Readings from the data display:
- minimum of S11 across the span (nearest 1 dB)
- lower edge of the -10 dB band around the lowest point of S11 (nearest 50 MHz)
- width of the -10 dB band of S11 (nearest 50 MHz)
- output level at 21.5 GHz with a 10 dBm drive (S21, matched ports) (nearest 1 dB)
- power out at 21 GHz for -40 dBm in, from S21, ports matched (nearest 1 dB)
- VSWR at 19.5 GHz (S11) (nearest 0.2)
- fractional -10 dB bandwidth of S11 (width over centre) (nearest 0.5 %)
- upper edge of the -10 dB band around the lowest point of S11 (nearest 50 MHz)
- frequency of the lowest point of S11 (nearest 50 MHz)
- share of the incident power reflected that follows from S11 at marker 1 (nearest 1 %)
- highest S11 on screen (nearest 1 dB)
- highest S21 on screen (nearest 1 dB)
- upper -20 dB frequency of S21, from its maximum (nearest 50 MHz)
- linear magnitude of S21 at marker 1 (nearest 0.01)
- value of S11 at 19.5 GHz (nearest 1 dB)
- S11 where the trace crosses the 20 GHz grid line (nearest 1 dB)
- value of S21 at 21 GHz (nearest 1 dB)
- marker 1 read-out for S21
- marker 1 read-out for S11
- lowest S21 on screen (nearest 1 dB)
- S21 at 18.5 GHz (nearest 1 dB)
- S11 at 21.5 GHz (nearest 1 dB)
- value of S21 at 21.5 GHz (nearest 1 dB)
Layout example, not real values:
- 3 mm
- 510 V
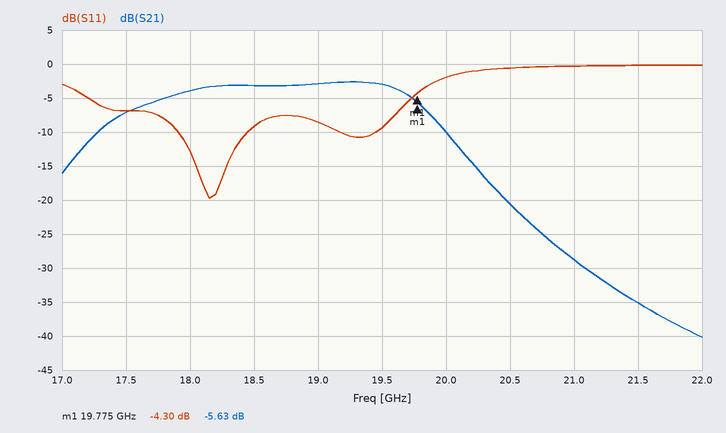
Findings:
- -20 dB
- 17.90 GHz
- 550 MHz
- -25 dBm
- -69 dBm
- 2.0
- 3.0 %
- 18.45 GHz
- 18.15 GHz
- 37 %
- 0 dB
- -3 dB
- 20.60 GHz
- 0.52
- -9 dB
- -2 dB
- -29 dB
- -5.63 dB
- -4.30 dB
- -40 dB
- -3 dB
- 0 dB
- -35 dB
